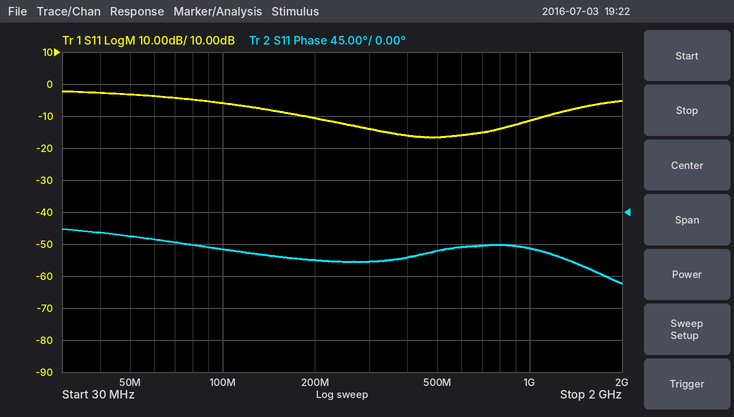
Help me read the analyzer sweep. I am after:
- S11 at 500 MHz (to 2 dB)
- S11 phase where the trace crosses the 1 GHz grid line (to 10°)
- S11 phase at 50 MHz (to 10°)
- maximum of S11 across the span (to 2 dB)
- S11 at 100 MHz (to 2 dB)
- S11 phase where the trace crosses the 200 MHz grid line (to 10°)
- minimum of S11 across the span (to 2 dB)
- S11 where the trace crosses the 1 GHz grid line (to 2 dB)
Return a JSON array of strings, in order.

["-16 dB", "-50°", "-30°", "-2 dB", "-6 dB", "-70°", "-16 dB", "-12 dB"]
